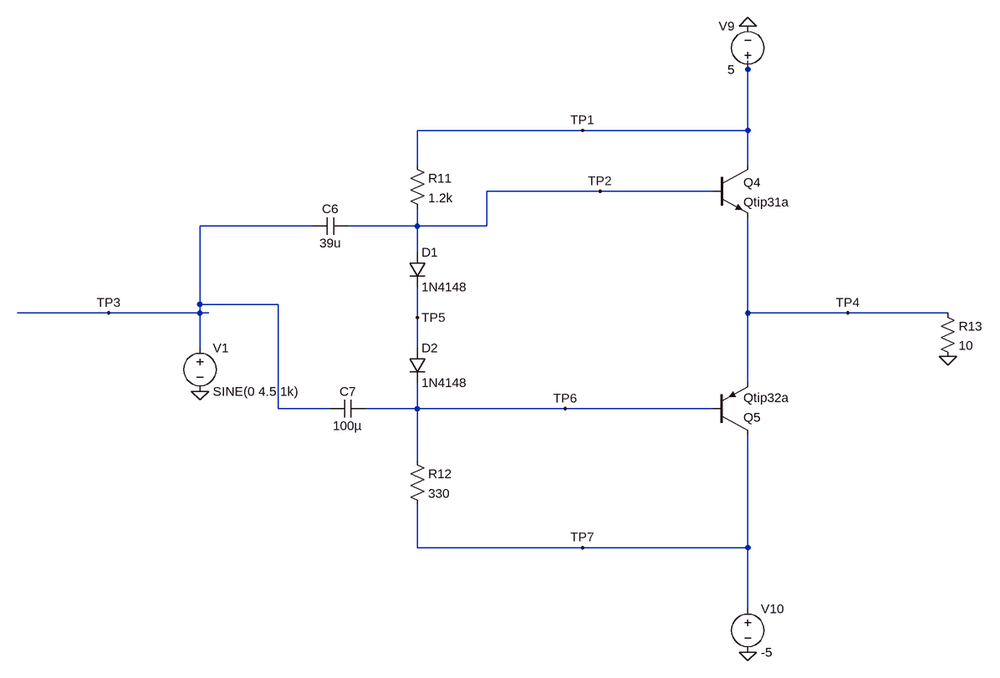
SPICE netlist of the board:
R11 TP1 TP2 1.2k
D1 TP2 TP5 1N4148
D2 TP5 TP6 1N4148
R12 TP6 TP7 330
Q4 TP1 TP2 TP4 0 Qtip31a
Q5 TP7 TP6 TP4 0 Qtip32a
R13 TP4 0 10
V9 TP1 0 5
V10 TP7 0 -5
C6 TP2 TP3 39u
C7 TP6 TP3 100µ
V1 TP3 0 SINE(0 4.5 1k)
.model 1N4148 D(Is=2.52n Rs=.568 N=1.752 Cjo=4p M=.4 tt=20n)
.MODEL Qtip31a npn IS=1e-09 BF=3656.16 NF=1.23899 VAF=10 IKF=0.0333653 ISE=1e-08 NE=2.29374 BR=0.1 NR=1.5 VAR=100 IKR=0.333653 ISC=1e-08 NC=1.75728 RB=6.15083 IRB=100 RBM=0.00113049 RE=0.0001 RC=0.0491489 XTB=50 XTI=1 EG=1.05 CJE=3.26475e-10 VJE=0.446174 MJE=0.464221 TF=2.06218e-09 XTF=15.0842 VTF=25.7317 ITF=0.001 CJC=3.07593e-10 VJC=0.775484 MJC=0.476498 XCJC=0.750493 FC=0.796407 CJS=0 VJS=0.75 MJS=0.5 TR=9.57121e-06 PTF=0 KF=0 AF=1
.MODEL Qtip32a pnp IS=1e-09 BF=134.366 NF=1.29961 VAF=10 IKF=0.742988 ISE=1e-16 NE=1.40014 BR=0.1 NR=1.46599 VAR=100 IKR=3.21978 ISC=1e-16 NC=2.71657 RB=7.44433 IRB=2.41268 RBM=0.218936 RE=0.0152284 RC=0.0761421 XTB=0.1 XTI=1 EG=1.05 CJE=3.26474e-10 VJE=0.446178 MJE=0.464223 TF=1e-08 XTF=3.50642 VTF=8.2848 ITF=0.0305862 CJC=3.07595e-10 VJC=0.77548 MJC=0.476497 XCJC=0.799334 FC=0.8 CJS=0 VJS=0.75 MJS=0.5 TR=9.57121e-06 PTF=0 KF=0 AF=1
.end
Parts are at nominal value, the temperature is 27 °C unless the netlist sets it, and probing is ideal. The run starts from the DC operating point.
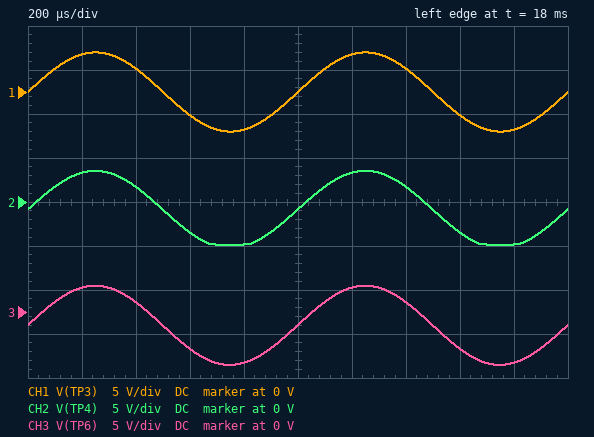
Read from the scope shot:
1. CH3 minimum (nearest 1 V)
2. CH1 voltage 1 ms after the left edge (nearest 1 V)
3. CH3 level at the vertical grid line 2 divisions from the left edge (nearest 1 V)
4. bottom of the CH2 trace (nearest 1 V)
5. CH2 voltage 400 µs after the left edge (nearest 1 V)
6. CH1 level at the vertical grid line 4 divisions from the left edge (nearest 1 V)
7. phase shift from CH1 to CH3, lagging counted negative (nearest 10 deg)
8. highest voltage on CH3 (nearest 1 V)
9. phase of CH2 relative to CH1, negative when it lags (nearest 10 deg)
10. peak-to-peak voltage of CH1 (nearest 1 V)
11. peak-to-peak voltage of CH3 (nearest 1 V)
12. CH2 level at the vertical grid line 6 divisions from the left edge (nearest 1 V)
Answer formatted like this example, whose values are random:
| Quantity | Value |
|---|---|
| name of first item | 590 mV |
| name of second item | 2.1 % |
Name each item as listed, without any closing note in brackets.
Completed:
| Quantity | Value |
|---|---|
| CH3 minimum | -6 V |
| CH1 voltage 1 ms after the left edge | 0 V |
| CH3 level at the vertical grid line 2 divisions from the left edge | 1 V |
| bottom of the CH2 trace | -5 V |
| CH2 voltage 400 µs after the left edge | 2 V |
| CH1 level at the vertical grid line 4 divisions from the left edge | -4 V |
| phase shift from CH1 to CH3, lagging counted negative | 0 deg |
| highest voltage on CH3 | 3 V |
| phase of CH2 relative to CH1, negative when it lags | 0 deg |
| peak-to-peak voltage of CH1 | 9 V |
| peak-to-peak voltage of CH3 | 9 V |
| CH2 level at the vertical grid line 6 divisions from the left edge | 3 V |
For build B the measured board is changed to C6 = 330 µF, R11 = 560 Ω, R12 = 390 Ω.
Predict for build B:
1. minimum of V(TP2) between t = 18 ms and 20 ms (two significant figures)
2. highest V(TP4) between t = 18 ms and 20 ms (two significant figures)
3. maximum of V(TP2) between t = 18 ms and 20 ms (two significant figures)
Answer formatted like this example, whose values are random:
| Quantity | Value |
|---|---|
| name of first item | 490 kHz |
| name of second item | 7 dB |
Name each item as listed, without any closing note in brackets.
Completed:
| Quantity | Value |
|---|---|
| minimum of V(TP2) between t = 18 ms and 20 ms | -4.3 V |
| highest V(TP4) between t = 18 ms and 20 ms | 4.0 V |
| maximum of V(TP2) between t = 18 ms and 20 ms | 4.7 V |
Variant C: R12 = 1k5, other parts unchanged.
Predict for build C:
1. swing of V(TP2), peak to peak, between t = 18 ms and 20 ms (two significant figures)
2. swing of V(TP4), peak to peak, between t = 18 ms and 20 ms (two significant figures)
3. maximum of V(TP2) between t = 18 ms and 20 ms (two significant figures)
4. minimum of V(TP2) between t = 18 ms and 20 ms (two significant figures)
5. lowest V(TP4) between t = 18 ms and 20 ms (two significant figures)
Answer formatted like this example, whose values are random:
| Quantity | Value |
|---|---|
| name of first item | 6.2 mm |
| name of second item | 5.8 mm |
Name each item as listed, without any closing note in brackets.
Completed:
| Quantity | Value |
|---|---|
| swing of V(TP2), peak to peak, between t = 18 ms and 20 ms | 9.0 V |
| swing of V(TP4), peak to peak, between t = 18 ms and 20 ms | 8.7 V |
| maximum of V(TP2) between t = 18 ms and 20 ms | 5.5 V |
| minimum of V(TP2) between t = 18 ms and 20 ms | -3.5 V |
| lowest V(TP4) between t = 18 ms and 20 ms | -4.0 V |
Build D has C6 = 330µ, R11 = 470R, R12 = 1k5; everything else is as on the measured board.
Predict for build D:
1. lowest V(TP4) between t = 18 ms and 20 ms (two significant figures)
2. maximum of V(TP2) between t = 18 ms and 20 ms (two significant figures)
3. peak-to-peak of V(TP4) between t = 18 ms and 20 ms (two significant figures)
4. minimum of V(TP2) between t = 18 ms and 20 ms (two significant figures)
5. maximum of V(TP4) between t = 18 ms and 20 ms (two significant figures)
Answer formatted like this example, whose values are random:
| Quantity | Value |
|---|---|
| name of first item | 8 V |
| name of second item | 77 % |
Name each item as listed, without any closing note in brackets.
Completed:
| Quantity | Value |
|---|---|
| lowest V(TP4) between t = 18 ms and 20 ms | -3.2 V |
| maximum of V(TP2) between t = 18 ms and 20 ms | 6.2 V |
| peak-to-peak of V(TP4) between t = 18 ms and 20 ms | 8.0 V |
| minimum of V(TP2) between t = 18 ms and 20 ms | -2.8 V |
| maximum of V(TP4) between t = 18 ms and 20 ms | 4.9 V |
